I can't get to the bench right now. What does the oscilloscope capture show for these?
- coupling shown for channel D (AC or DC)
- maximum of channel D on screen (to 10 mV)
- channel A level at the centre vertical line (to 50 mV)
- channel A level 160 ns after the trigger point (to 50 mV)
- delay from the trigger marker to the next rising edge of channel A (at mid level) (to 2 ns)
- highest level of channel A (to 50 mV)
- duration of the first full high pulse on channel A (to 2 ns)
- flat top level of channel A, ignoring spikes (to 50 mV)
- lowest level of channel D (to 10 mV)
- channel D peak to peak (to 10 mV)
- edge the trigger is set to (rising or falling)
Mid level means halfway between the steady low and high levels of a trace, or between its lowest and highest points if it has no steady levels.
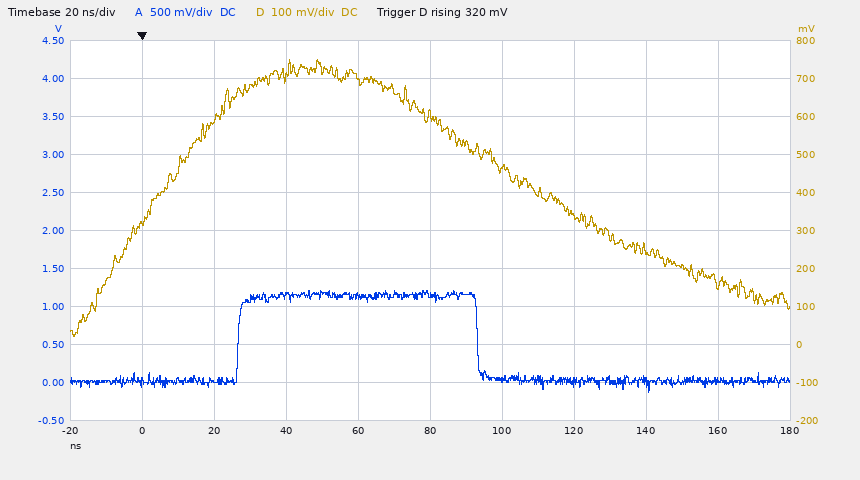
DC
750 mV
1.15 V
0 mV
26 ns
1.20 V
66 ns
1.15 V
20 mV
730 mV
rising
